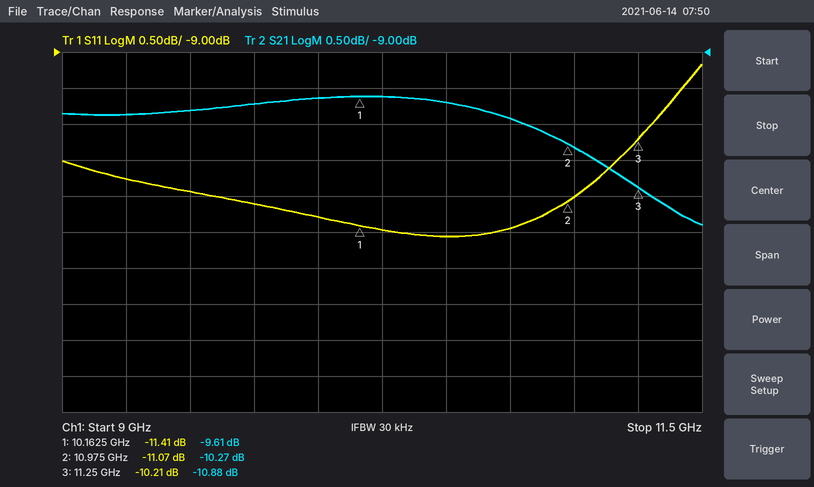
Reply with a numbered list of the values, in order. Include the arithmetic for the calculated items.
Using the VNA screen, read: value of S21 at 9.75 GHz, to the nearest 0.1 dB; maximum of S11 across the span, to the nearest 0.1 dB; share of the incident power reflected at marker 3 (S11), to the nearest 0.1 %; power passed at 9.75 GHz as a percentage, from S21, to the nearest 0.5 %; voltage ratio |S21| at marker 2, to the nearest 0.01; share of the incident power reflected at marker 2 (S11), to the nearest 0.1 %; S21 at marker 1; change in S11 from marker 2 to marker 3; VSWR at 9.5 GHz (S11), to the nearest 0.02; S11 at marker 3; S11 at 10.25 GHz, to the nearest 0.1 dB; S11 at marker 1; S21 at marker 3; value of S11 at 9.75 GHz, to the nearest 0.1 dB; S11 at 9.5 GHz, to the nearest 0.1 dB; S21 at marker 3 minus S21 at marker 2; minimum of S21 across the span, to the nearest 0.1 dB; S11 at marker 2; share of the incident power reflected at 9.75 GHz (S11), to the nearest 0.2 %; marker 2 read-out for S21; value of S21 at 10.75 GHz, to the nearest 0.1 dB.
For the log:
1. -9.7 dB
2. -9.2 dB
3. 10^(-10.21/10) ≈ 9.5 %
4. 10^(-9.7/10) ≈ 10.7 %, so 10.5 % to the nearest 0.5 %
5. 10^(-10.27/20) ≈ 0.31
6. 10^(-11.07/10) ≈ 7.8 %
7. -9.61 dB
8. -10.21 − (-11.07) = 0.86 dB
9. |Γ| = 10^(-10.9/20) = 0.2851; VSWR = (1 + 0.2851)/(1 − 0.2851) ≈ 1.80
10. -10.21 dB
11. -11.5 dB
12. -11.41 dB
13. -10.88 dB
14. -11.1 dB
15. -10.9 dB
16. -10.88 − (-10.27) = -0.61 dB
17. -11.4 dB
18. -11.07 dB
19. 10^(-11.1/10) ≈ 7.8 %
20. -10.27 dB
21. -9.9 dB
